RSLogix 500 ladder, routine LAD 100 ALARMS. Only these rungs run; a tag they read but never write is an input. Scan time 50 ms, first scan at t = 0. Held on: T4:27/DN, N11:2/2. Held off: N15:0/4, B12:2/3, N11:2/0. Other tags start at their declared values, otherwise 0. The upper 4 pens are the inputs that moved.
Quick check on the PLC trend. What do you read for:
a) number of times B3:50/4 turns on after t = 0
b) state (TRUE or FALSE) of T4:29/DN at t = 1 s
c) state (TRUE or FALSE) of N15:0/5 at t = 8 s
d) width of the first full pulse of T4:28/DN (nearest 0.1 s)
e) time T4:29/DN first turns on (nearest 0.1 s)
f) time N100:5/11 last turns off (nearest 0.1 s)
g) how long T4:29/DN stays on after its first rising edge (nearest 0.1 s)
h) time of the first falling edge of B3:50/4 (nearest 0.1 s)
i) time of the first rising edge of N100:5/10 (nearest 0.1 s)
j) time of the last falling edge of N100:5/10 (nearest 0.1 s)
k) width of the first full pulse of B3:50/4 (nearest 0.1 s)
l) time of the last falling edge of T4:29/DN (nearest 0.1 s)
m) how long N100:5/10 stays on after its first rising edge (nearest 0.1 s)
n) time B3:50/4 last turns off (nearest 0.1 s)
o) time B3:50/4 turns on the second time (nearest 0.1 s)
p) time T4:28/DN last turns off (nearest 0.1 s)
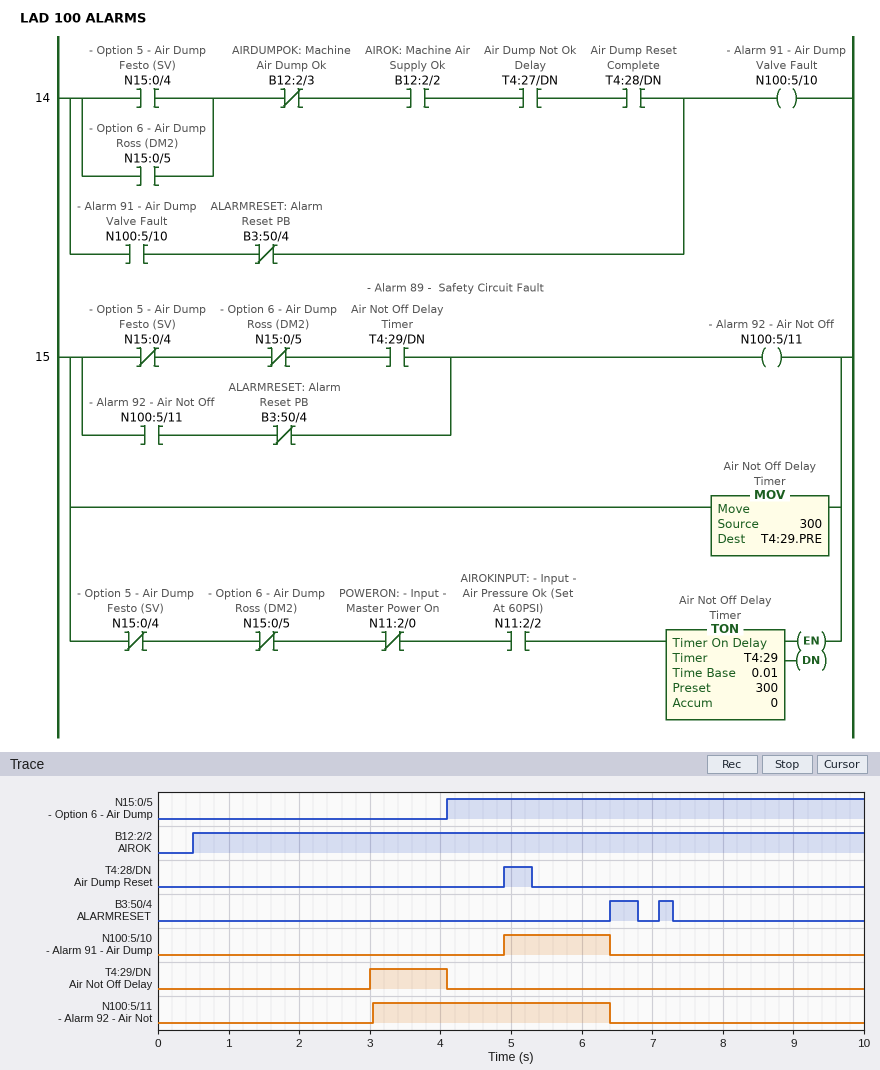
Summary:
2
FALSE
TRUE
0.4 s
3.0 s
6.4 s
1.1 s
6.8 s
4.9 s
6.4 s
0.4 s
4.1 s
1.5 s
7.3 s
7.1 s
5.3 s
